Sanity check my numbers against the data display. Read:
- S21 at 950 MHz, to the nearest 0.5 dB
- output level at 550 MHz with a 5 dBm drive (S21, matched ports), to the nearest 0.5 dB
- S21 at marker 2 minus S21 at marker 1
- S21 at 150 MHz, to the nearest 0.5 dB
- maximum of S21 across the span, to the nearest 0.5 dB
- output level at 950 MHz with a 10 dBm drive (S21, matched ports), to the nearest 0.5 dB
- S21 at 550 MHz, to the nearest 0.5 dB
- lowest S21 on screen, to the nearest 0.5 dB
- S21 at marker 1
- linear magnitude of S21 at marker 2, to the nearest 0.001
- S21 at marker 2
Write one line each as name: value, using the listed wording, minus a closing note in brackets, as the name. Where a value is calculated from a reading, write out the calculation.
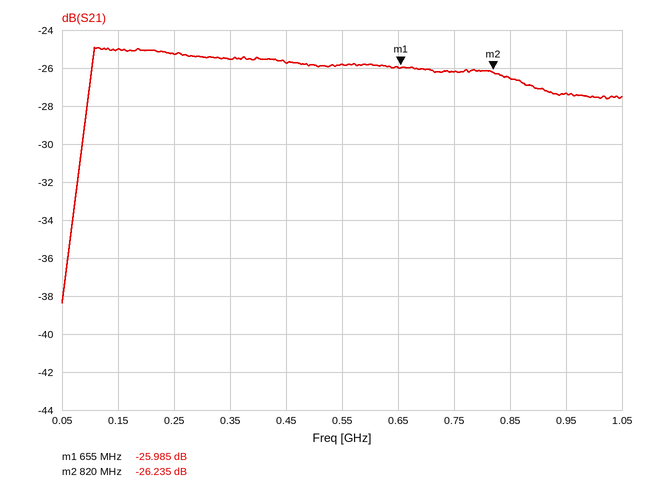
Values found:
S21 at 950 MHz, to the nearest 0.5 dB: -27.5 dB
output level at 550 MHz with a 5 dBm drive (S21, matched ports), to the nearest 0.5 dB: 5 dBm + (-26.0 dB) = -21.0 dBm
S21 at marker 2 minus S21 at marker 1: -26.235 − (-25.985) = -0.250 dB
S21 at 150 MHz, to the nearest 0.5 dB: -25.0 dB
maximum of S21 across the span, to the nearest 0.5 dB: -25.0 dB
output level at 950 MHz with a 10 dBm drive (S21, matched ports), to the nearest 0.5 dB: 10 dBm + (-27.5 dB) = -17.5 dBm
S21 at 550 MHz, to the nearest 0.5 dB: -26.0 dB
lowest S21 on screen, to the nearest 0.5 dB: -38.5 dB
S21 at marker 1: -25.985 dB
linear magnitude of S21 at marker 2, to the nearest 0.001: 10^(-26.235/20) ≈ 0.049
S21 at marker 2: -26.235 dB
